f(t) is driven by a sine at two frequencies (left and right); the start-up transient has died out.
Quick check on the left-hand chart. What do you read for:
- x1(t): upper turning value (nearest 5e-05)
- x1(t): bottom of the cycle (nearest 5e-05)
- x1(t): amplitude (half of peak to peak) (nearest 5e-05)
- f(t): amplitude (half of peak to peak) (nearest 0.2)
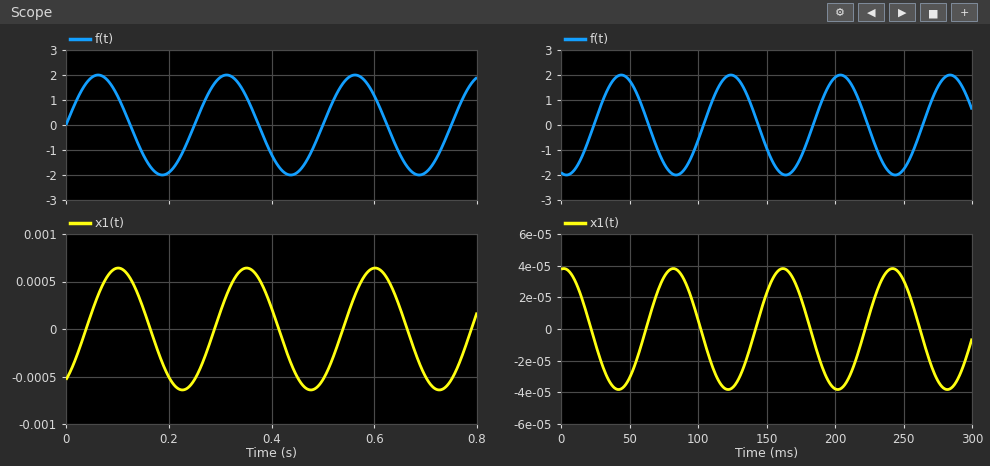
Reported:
0.00065
-0.00065
0.00065
2.0
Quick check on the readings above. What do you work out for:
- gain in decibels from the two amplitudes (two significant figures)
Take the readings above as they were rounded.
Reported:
-70 dB
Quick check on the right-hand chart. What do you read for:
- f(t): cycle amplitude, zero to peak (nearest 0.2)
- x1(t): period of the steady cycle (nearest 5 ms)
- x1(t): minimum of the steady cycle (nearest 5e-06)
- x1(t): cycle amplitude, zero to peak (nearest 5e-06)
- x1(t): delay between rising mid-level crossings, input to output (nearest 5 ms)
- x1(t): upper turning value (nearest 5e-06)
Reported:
2.0
80 ms
-0.000040
0.000040
40 ms
0.000040
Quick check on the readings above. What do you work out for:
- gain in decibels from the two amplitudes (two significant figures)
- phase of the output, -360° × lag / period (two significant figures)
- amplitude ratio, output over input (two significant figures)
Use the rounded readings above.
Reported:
-94 dB
-180°
0.000020
